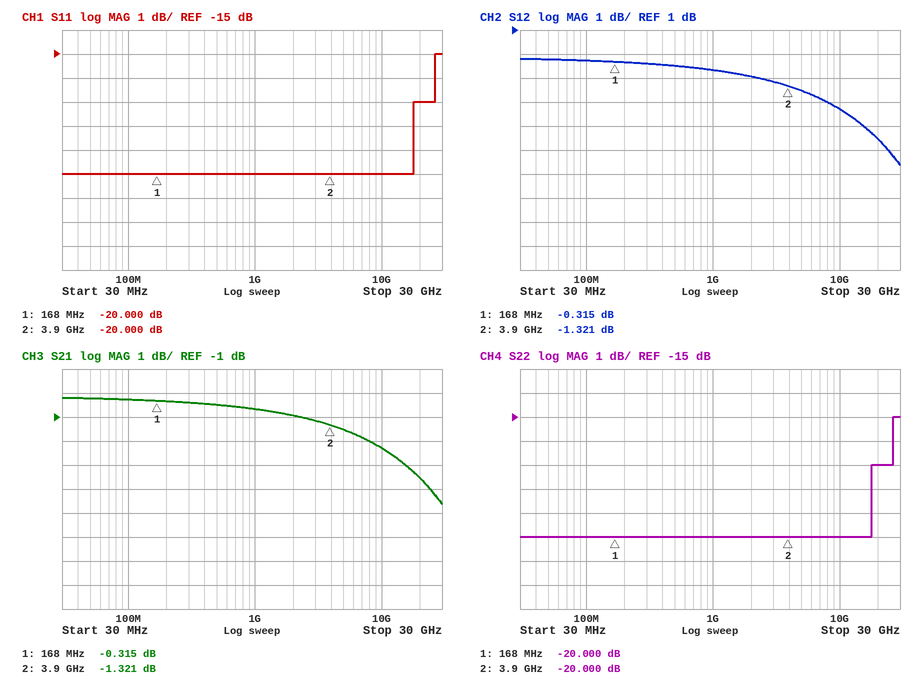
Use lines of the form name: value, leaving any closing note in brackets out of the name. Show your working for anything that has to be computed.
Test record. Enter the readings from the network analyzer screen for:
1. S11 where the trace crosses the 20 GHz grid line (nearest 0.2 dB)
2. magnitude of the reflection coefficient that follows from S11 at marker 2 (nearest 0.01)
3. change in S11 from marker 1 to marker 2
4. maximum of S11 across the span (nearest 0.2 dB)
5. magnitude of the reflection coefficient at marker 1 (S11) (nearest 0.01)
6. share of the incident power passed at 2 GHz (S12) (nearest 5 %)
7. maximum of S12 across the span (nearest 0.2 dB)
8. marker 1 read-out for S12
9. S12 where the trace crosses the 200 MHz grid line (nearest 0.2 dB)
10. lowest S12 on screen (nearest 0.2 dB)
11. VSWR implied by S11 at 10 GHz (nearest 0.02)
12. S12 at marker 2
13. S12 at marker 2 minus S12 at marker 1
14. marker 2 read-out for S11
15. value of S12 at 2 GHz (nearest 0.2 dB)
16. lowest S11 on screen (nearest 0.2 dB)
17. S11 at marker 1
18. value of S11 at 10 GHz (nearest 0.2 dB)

S11 where the trace crosses the 20 GHz grid line: -17.0 dB
magnitude of the reflection coefficient that follows from S11 at marker 2: 10^(-20/20) ≈ 0.10
change in S11 from marker 1 to marker 2: -20 − (-20) = 0.000 dB
maximum of S11 across the span: -15.0 dB
magnitude of the reflection coefficient at marker 1 (S11): 10^(-20/20) ≈ 0.10
share of the incident power passed at 2 GHz (S12): 10^(-1/10) ≈ 79.4 %, so 80 % to the nearest 5 %
maximum of S12 across the span: -0.2 dB
marker 1 read-out for S12: -0.315 dB
S12 where the trace crosses the 200 MHz grid line: -0.4 dB
lowest S12 on screen: -4.6 dB
VSWR implied by S11 at 10 GHz: |Γ| = 10^(-20/20) = 0.1000; VSWR = (1 + 0.1000)/(1 − 0.1000) ≈ 1.22
S12 at marker 2: -1.321 dB
S12 at marker 2 minus S12 at marker 1: -1.321 − (-0.315) = -1.006 dB
marker 2 read-out for S11: -20.000 dB
value of S12 at 2 GHz: -1.0 dB
lowest S11 on screen: -20.0 dB
S11 at marker 1: -20.000 dB
value of S11 at 10 GHz: -20.0 dB
